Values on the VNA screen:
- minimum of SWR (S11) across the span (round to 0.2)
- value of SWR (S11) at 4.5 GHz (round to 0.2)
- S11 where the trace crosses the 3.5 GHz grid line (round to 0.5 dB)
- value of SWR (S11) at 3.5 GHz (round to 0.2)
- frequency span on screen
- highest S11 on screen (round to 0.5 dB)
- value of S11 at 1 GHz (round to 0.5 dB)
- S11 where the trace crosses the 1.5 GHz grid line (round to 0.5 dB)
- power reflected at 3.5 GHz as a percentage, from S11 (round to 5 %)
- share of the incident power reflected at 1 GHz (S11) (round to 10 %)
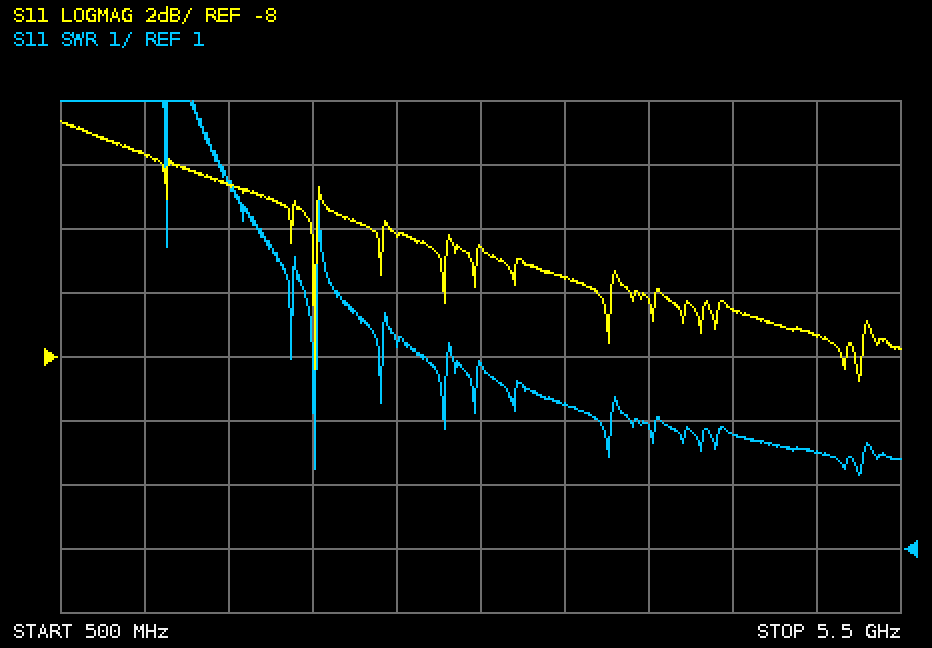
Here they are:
2.2
2.8
-5.5 dB
3.2
5 GHz
-0.5 dB
-1.5 dB
-2.5 dB
30 %
70 %
